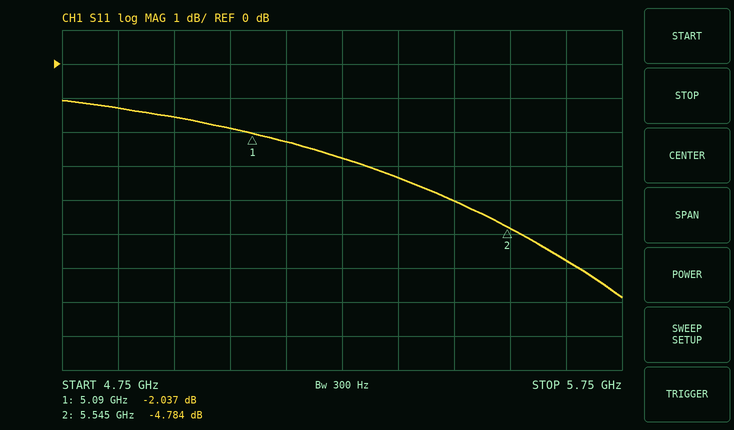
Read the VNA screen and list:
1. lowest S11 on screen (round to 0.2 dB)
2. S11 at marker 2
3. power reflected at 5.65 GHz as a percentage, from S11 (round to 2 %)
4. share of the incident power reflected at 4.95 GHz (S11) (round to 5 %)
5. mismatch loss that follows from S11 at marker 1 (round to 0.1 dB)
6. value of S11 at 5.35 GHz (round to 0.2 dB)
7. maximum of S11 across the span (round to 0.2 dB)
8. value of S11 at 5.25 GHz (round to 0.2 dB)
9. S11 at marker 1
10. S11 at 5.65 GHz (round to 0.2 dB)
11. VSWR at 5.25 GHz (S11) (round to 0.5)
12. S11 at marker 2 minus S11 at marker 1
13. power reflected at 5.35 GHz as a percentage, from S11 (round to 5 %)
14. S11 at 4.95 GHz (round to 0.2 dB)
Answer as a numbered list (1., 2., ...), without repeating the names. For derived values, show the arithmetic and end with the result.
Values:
1. -6.8 dB
2. -4.784 dB
3. 10^(-5.8/10) ≈ 26 %
4. 10^(-1.6/10) ≈ 69.2 %, so 70 % to the nearest 5 %
5. −10 log10(1 − 10^(-2.037/10)) ≈ 4.3 dB
6. -3.4 dB
7. -1.0 dB
8. -2.8 dB
9. -2.037 dB
10. -5.8 dB
11. |Γ| = 10^(-2.8/20) = 0.7244; VSWR = (1 + 0.7244)/(1 − 0.7244) ≈ 6.26, so 6.5 to the nearest 0.5
12. -4.784 − (-2.037) = -2.747 dB
13. 10^(-3.4/10) ≈ 45.7 %, so 45 % to the nearest 5 %
14. -1.6 dB
